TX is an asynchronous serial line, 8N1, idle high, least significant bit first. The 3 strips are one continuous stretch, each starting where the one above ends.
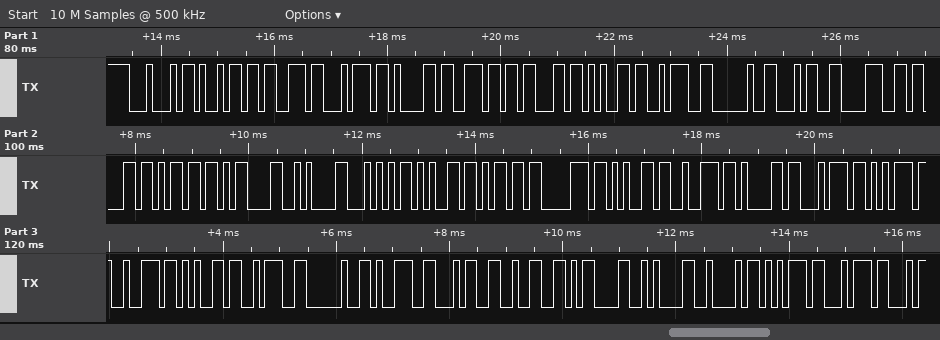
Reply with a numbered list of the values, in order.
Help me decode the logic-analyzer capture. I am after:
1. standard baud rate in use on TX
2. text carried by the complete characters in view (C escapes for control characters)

1. 9600 baud
2. "Distance: 48cm\r\nTemperature: 942\r\nBut"
